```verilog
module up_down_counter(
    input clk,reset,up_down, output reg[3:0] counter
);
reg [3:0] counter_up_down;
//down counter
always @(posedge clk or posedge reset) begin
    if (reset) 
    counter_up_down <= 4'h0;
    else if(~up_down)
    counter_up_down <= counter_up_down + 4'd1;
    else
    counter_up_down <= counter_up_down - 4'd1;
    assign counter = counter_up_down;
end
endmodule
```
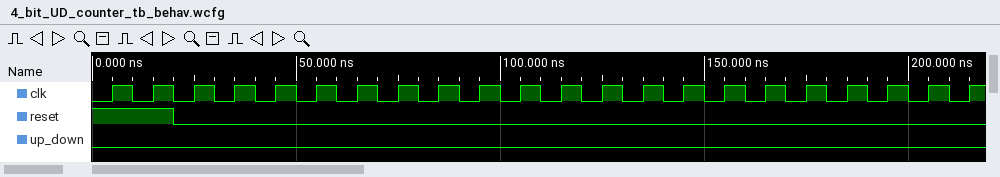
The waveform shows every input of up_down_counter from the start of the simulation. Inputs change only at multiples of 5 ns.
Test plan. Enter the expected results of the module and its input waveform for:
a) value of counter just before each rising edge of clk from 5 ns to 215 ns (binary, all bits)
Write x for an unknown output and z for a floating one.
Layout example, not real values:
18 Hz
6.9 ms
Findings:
0000, 0000, 0000, 0001, 0010, 0011, 0100, 0101, 0110, 0111, 1000, 1001, 1010, 1011, 1100, 1101, 1110, 1111, 0000, 0001, 0010, 0011
